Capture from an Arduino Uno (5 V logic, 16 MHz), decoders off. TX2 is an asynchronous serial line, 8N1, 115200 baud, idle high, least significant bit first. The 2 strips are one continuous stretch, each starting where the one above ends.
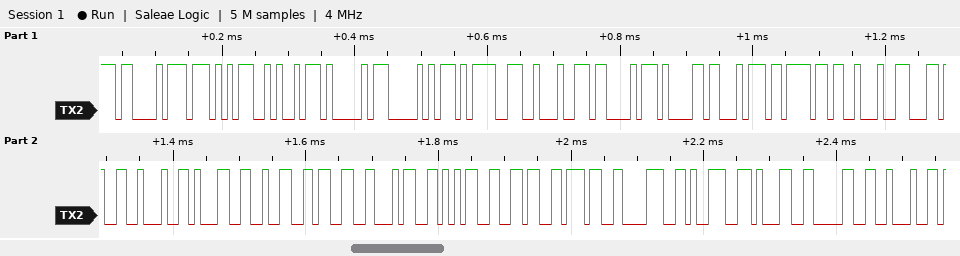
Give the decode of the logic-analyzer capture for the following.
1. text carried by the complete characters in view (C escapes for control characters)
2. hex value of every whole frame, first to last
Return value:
"CWJAP=\"Cato\",\"12345678910\""
43 57 4A 41 50 3D 22 43 61 74 6F 22 2C 22 31 32 33 34 35 36 37 38 39 31 30 22
